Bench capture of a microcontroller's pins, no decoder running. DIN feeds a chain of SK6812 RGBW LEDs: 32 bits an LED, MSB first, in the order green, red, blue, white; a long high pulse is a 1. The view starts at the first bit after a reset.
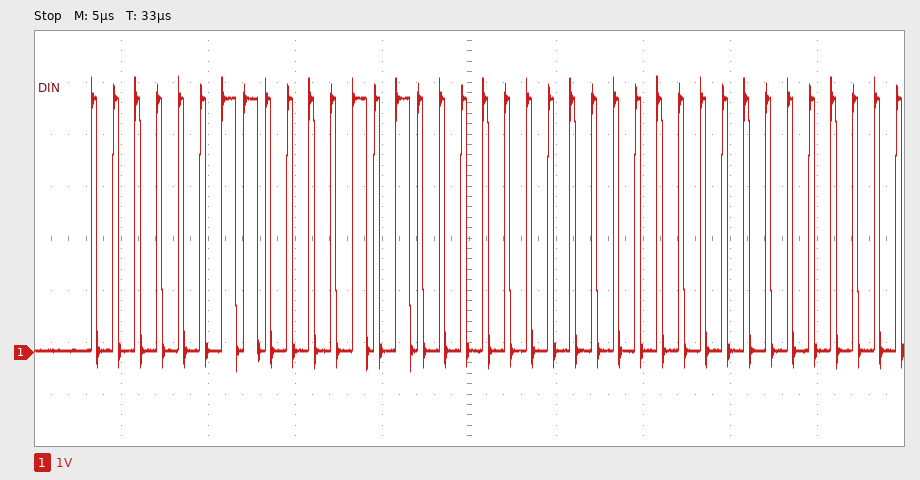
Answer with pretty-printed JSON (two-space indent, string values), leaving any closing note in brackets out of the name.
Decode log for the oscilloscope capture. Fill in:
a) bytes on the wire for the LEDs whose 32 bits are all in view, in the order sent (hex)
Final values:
{
  "bytes on the wire for the LEDs whose 32 bits are all in view, in the order sent": "03 0A 00 00"
}
